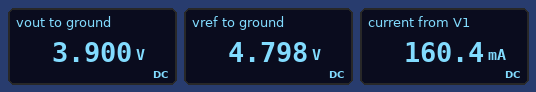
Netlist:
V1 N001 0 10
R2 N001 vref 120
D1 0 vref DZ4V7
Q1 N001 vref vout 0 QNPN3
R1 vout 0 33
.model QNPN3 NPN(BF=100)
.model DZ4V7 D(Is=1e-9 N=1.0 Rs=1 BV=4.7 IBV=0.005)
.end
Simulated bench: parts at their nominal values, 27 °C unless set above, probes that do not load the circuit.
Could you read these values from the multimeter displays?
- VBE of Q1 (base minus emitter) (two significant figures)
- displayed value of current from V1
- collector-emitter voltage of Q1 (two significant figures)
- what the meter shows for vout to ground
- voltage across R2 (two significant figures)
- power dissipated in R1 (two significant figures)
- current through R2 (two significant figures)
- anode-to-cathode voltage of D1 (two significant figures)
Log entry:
900 mV
160.4 mA
6.1 V
3.900 V
5.2 V
460 mW
43 mA
-4.8 V
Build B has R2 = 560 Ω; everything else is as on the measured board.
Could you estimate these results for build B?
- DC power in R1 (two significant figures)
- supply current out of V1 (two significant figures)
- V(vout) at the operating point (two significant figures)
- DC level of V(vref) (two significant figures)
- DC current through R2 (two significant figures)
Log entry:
440 mW
120 mA
3.8 V
4.7 V
9.4 mA
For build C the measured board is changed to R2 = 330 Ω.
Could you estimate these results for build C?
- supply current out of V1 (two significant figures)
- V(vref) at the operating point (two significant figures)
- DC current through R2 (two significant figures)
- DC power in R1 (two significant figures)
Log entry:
130 mA
4.7 V
16 mA
450 mW
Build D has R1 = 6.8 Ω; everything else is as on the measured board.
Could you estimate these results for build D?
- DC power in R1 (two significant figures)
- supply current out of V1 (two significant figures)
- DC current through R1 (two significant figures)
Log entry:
2.2 W
600 mA
570 mA
